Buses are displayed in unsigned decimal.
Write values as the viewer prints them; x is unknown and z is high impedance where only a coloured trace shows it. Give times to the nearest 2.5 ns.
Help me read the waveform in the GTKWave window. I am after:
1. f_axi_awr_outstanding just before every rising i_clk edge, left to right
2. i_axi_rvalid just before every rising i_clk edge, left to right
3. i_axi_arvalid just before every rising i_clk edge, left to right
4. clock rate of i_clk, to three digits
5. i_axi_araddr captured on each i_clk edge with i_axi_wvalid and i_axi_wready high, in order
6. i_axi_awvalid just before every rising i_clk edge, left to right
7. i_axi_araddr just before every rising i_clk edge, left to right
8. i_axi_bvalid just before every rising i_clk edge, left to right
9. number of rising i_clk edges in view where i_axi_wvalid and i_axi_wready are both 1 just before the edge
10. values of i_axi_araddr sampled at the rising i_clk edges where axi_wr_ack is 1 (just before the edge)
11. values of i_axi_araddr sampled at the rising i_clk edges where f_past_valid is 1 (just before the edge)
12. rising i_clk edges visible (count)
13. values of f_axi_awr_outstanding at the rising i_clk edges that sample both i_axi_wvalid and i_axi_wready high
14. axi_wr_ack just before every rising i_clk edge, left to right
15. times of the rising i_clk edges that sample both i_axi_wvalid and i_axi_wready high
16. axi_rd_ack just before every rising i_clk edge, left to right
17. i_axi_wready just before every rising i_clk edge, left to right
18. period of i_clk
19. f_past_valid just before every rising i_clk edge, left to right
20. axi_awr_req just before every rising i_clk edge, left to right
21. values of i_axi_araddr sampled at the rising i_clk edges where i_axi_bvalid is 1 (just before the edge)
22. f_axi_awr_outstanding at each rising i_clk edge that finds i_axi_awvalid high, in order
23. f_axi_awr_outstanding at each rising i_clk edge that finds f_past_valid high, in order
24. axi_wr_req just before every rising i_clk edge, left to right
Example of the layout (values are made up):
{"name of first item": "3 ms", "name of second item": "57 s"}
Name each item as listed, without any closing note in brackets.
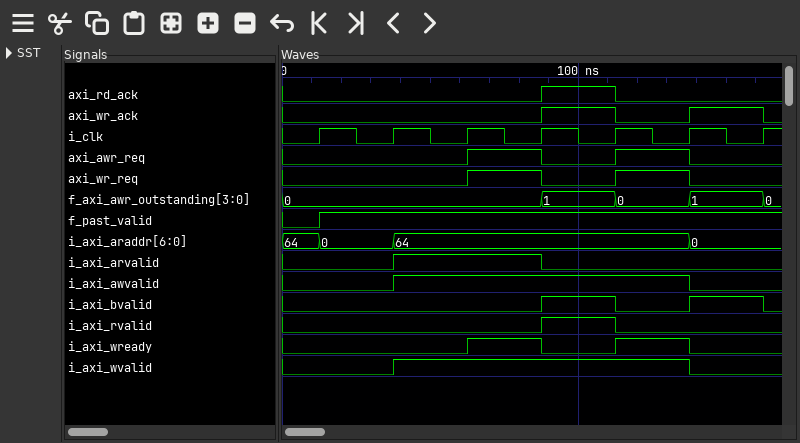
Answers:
{"f_axi_awr_outstanding just before every rising i_clk edge, left to right": "0, 0, 0, 0, 1, 0, 1", "i_axi_rvalid just before every rising i_clk edge, left to right": "0 0 0 0 1 0 0", "i_axi_arvalid just before every rising i_clk edge, left to right": "0 0 1 1 0 0 0", "clock rate of i_clk, to three digits": "40.0 MHz", "i_axi_araddr captured on each i_clk edge with i_axi_wvalid and i_axi_wready high, in order": "64, 64", "i_axi_awvalid just before every rising i_clk edge, left to right": "0 0 1 1 1 1 0", "i_axi_araddr just before every rising i_clk edge, left to right": "64, 0, 64, 64, 64, 64, 0", "i_axi_bvalid just before every rising i_clk edge, left to right": "0 0 0 0 1 0 1", "number of rising i_clk edges in view where i_axi_wvalid and i_axi_wready are both 1 just before the edge": "2", "values of i_axi_araddr sampled at the rising i_clk edges where axi_wr_ack is 1": "64, 0", "values of i_axi_araddr sampled at the rising i_clk edges where f_past_valid is 1": "0, 64, 64, 64, 64, 0", "rising i_clk edges visible": "7", "values of f_axi_awr_outstanding at the rising i_clk edges that sample both i_axi_wvalid and i_axi_wready high": "0, 0", "axi_wr_ack just before every rising i_clk edge, left to right": "0 0 0 0 1 0 1", "times of the rising i_clk edges that sample both i_axi_wvalid and i_axi_wready high": "87.5 ns, 137.5 ns", "axi_rd_ack just before every rising i_clk edge, left to right": "0 0 0 0 1 0 0", "i_axi_wready just before every rising i_clk edge, left to right": "0 0 0 1 0 1 0", "period of i_clk": "25 ns", "f_past_valid just before every rising i_clk edge, left to right": "0 1 1 1 1 1 1", "axi_awr_req just before every rising i_clk edge, left to right": "0 0 0 1 0 1 0", "values of i_axi_araddr sampled at the rising i_clk edges where i_axi_bvalid is 1": "64, 0", "f_axi_awr_outstanding at each rising i_clk edge that finds i_axi_awvalid high, in order": "0, 0, 1, 0", "f_axi_awr_outstanding at each rising i_clk edge that finds f_past_valid high, in order": "0, 0, 0, 1, 0, 1", "axi_wr_req just before every rising i_clk edge, left to right": "0 0 0 1 0 1 0"}
